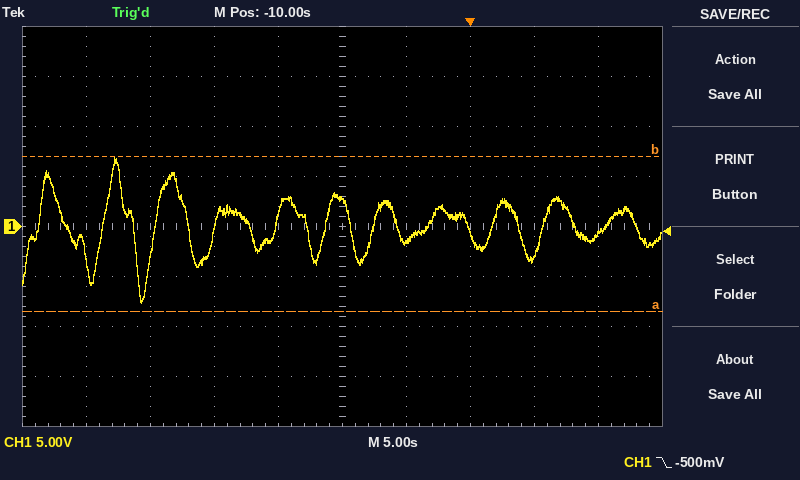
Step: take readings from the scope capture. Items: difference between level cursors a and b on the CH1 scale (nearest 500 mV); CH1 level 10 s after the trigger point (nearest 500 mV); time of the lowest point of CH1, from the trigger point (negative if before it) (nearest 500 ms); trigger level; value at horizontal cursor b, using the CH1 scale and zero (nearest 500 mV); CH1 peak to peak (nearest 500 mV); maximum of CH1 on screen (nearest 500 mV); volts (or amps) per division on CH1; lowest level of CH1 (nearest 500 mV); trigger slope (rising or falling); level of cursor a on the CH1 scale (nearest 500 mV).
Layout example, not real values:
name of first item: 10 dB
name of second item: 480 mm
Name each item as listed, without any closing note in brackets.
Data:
difference between level cursors a and b on the CH1 scale: 15.5 V
CH1 level 10 s after the trigger point: -500 mV
time of the lowest point of CH1, from the trigger point (negative if before it): -25.5 s
trigger level: -500 mV
value at horizontal cursor b, using the CH1 scale and zero: 7.0 V
CH1 peak to peak: 14.5 V
maximum of CH1 on screen: 7.0 V
volts (or amps) per division on CH1: 5 V
lowest level of CH1: -7.5 V
trigger slope: falling
level of cursor a on the CH1 scale: -8.5 V
